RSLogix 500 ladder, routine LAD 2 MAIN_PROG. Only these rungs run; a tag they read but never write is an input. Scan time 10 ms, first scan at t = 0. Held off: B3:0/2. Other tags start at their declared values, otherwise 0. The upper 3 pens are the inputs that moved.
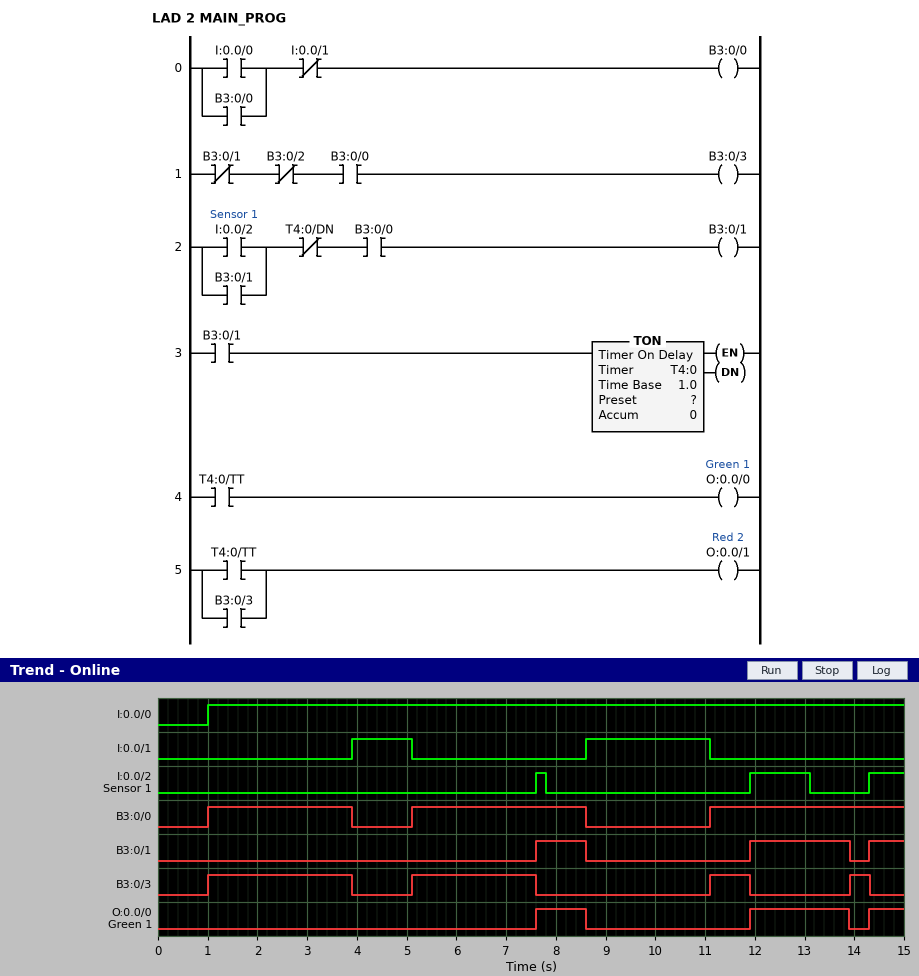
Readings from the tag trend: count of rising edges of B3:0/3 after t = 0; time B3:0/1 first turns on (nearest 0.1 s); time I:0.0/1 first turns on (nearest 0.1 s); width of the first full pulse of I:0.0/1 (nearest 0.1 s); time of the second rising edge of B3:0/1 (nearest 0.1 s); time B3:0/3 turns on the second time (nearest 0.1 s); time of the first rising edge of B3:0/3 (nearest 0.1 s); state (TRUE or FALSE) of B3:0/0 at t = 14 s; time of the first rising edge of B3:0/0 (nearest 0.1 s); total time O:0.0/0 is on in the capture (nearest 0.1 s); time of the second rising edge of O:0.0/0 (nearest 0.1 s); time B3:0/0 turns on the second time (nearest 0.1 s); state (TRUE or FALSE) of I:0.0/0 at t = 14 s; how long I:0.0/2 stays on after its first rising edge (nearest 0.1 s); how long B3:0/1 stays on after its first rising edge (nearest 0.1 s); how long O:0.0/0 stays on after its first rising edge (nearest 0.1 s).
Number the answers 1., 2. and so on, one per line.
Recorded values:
1. 4
2. 7.6 s
3. 3.9 s
4. 1.2 s
5. 11.9 s
6. 5.1 s
7. 1.0 s
8. TRUE
9. 1.0 s
10. 3.7 s
11. 11.9 s
12. 5.1 s
13. TRUE
14. 0.2 s
15. 1.0 s
16. 1.0 s
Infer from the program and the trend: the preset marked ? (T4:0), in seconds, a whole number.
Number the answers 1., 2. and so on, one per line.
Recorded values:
1. 2 s
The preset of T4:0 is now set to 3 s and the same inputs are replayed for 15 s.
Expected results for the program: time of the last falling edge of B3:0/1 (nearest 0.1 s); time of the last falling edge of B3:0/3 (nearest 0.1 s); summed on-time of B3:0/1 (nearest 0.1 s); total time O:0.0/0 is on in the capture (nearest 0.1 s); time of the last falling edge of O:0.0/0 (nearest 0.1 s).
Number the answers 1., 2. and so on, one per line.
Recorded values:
1. 14.9 s
2. 14.9 s
3. 4.1 s
4. 4.1 s
5. 14.9 s
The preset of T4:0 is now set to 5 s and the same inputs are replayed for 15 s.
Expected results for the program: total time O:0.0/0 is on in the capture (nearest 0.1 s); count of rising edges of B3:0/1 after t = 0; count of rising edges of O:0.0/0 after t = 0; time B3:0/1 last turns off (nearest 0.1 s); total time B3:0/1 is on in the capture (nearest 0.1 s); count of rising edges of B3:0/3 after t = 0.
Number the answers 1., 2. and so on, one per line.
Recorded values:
1. 4.1 s
2. 2
3. 2
4. 8.6 s
5. 4.1 s
6. 3
